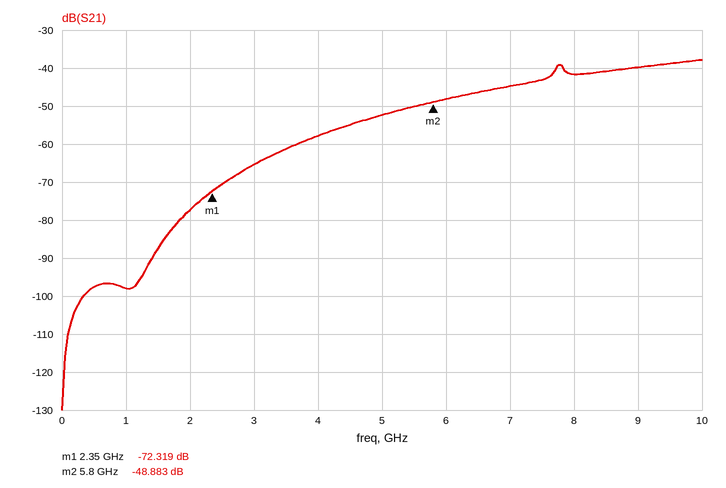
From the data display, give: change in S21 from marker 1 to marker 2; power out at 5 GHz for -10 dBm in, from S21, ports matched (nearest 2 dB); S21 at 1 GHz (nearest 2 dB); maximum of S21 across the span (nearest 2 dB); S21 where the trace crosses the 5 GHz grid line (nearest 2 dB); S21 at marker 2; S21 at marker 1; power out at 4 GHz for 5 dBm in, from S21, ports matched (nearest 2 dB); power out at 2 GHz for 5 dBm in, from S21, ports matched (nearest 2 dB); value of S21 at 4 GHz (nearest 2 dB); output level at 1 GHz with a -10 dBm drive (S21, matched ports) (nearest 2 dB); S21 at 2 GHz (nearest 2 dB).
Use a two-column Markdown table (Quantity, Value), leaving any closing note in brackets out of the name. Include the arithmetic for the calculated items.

| Quantity | Value |
|---|---|
| change in S21 from marker 1 to marker 2 | -48.883 − (-72.319) = 23.436 dB |
| power out at 5 GHz for -10 dBm in, from S21, ports matched | -10 dBm + (-52 dB) = -62 dBm |
| S21 at 1 GHz | -98 dB |
| maximum of S21 across the span | -38 dB |
| S21 where the trace crosses the 5 GHz grid line | -52 dB |
| S21 at marker 2 | -48.883 dB |
| S21 at marker 1 | -72.319 dB |
| power out at 4 GHz for 5 dBm in, from S21, ports matched | 5 dBm + (-58 dB) = -52 dBm |
| power out at 2 GHz for 5 dBm in, from S21, ports matched | 5 dBm + (-78 dB) = -72 dBm |
| value of S21 at 4 GHz | -58 dB |
| output level at 1 GHz with a -10 dBm drive (S21, matched ports) | -10 dBm + (-98 dB) = -108 dBm |
| S21 at 2 GHz | -78 dB |
